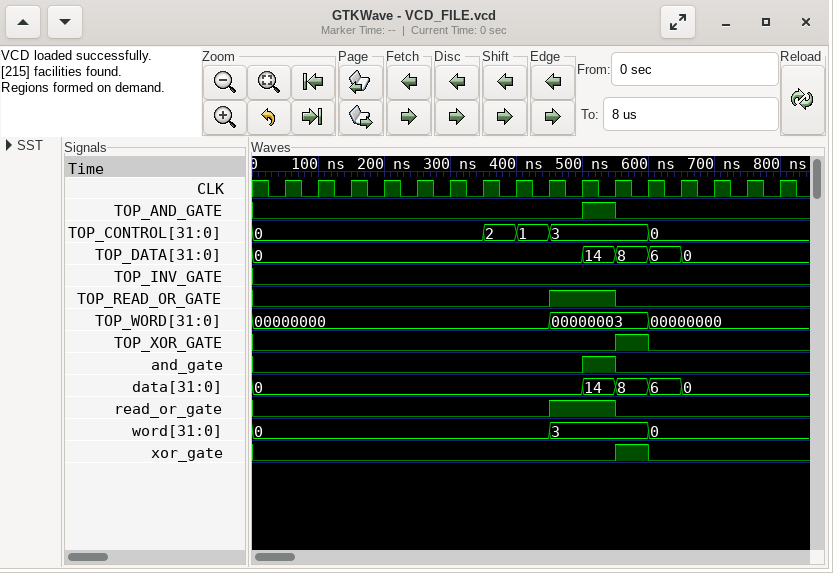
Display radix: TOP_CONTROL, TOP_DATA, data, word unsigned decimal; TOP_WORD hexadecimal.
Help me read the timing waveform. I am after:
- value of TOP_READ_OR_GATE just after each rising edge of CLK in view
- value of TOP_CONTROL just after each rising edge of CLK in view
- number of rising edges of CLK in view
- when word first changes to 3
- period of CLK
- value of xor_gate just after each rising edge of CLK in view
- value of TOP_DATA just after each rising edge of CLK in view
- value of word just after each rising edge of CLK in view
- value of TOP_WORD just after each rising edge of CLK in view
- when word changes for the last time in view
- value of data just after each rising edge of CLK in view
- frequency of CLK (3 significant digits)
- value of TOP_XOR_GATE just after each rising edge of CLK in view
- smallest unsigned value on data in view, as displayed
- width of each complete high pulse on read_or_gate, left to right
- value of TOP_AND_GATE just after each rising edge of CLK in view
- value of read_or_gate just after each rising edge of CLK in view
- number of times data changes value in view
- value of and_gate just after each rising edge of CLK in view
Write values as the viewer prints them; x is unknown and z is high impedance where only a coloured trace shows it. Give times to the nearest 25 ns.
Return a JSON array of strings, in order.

["0 0 0 0 0 0 0 0 1 1 0 0 0 0 0 0", "0, 0, 0, 0, 0, 0, 2, 1, 3, 3, 3, 0, 0, 0, 0, 0", "16", "450 ns", "50 ns", "0 0 0 0 0 0 0 0 0 0 1 0 0 0 0 0", "0, 0, 0, 0, 0, 0, 0, 0, 0, 14, 8, 6, 0, 0, 0, 0", "0, 0, 0, 0, 0, 0, 0, 0, 3, 3, 3, 0, 0, 0, 0, 0", "00000000, 00000000, 00000000, 00000000, 00000000, 00000000, 00000000, 00000000, 00000003, 00000003, 00000003, 00000000, 00000000, 00000000, 00000000, 00000000", "600 ns", "0, 0, 0, 0, 0, 0, 0, 0, 0, 14, 8, 6, 0, 0, 0, 0", "20.0 MHz", "0 0 0 0 0 0 0 0 0 0 1 0 0 0 0 0", "0", "100 ns", "0 0 0 0 0 0 0 0 0 1 0 0 0 0 0 0", "0 0 0 0 0 0 0 0 1 1 0 0 0 0 0 0", "4", "0 0 0 0 0 0 0 0 0 1 0 0 0 0 0 0"]
